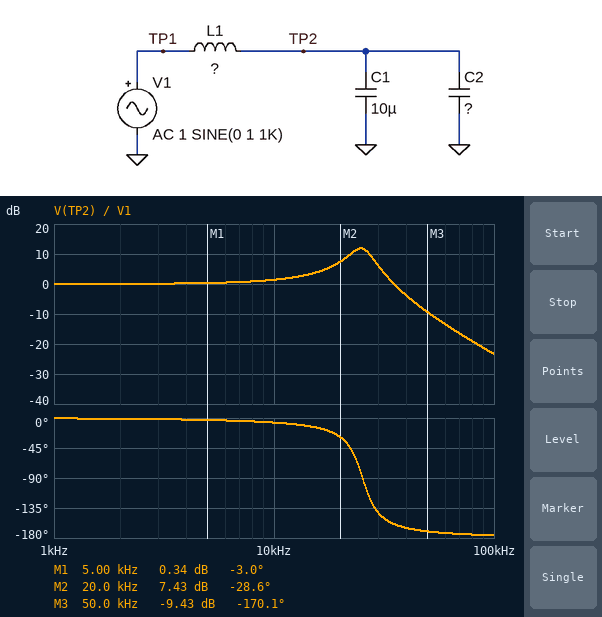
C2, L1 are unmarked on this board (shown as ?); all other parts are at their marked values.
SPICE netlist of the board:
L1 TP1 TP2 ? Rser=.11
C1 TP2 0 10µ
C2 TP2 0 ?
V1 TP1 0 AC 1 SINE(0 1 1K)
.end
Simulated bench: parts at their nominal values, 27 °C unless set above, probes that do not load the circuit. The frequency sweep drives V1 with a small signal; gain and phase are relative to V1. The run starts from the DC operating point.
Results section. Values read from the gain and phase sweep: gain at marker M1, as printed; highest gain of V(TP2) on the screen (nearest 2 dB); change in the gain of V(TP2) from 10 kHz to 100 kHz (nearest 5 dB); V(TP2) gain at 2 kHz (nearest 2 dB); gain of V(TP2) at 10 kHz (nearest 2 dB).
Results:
0.34 dB
12 dB
-25 dB
0 dB
2 dB
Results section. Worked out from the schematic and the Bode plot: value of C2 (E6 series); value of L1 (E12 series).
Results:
4.7 µF
2.7 µH
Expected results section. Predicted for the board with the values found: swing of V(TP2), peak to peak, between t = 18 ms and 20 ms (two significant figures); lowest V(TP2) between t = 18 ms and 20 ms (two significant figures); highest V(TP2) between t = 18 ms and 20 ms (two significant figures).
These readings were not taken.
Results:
2.0 V
-1.0 V
1.0 V
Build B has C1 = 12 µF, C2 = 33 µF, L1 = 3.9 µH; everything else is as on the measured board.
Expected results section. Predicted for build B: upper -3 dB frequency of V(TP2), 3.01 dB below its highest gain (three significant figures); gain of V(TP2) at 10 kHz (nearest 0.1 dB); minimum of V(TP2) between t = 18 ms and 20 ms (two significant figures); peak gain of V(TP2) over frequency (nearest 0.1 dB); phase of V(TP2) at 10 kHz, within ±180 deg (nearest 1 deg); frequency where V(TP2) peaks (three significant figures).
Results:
13.7 kHz
7.2 dB
-1.0 V
8.7 dB
-45 deg
11.6 kHz
